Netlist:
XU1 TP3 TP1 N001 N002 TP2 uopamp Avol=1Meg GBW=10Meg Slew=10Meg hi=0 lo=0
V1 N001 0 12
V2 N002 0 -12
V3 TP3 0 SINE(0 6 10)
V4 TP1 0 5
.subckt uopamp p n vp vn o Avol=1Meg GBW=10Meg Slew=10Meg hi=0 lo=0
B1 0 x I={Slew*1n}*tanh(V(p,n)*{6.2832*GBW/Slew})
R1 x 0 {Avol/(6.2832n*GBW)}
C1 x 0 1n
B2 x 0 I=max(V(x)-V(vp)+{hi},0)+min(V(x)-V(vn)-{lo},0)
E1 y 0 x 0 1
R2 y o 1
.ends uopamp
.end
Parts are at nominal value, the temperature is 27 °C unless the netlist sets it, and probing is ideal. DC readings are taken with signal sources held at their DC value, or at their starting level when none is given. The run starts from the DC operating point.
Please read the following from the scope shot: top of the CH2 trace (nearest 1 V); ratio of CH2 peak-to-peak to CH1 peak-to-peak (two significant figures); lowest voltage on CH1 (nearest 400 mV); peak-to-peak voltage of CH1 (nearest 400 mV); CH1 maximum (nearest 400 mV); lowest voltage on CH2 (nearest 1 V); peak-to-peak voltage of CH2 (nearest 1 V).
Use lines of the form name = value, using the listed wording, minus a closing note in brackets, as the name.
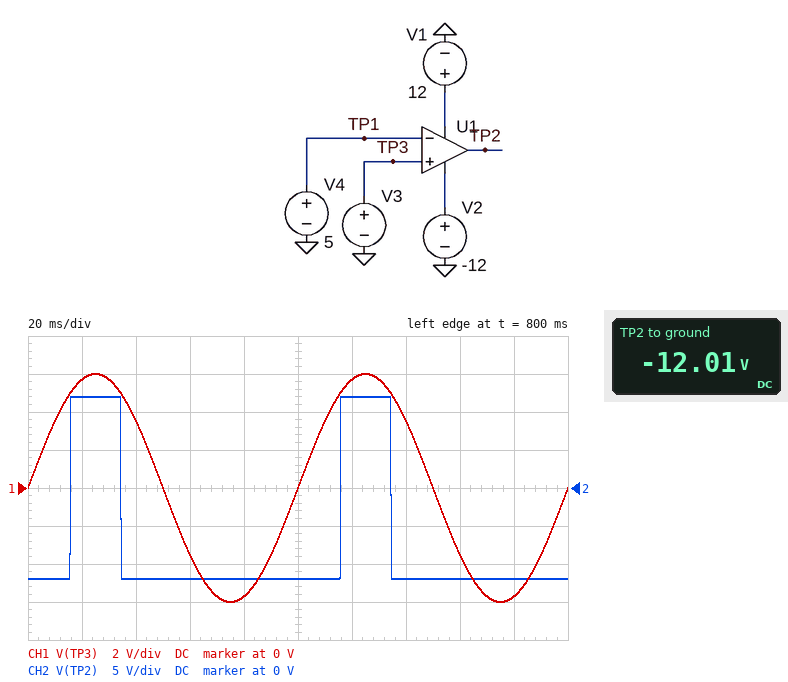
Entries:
top of the CH2 trace = 12 V
ratio of CH2 peak-to-peak to CH1 peak-to-peak = 2.0
lowest voltage on CH1 = -6.0 V
peak-to-peak voltage of CH1 = 12.0 V
CH1 maximum = 6.0 V
lowest voltage on CH2 = -12 V
peak-to-peak voltage of CH2 = 24 V
